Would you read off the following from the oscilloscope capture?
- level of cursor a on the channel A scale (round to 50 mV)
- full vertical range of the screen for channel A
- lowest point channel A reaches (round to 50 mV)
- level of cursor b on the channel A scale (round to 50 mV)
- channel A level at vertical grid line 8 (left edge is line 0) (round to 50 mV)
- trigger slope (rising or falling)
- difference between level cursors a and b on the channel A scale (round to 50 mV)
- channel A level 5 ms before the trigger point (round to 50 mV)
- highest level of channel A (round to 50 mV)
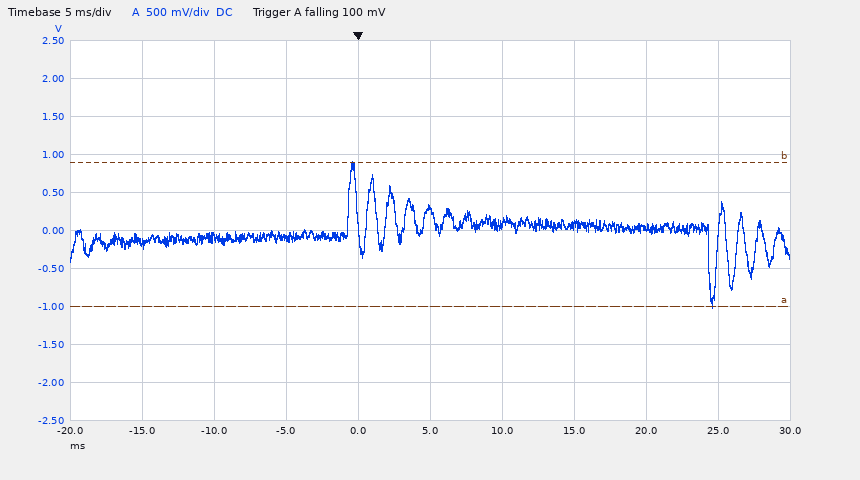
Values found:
-1.00 V
5 V
-1.00 V
900 mV
50 mV
falling
1.90 V
-100 mV
900 mV
